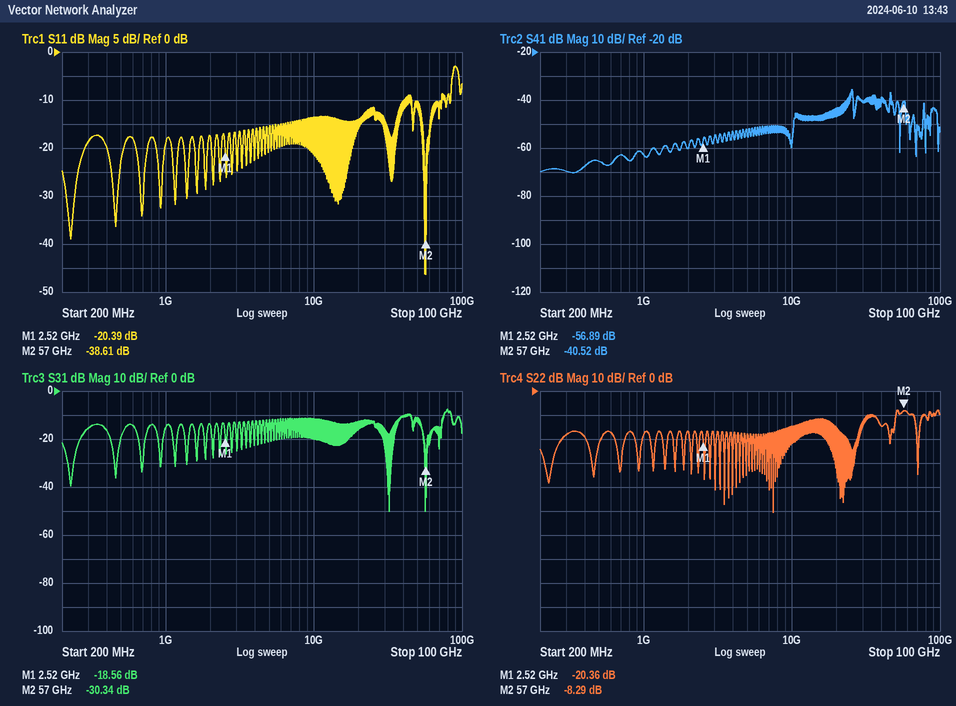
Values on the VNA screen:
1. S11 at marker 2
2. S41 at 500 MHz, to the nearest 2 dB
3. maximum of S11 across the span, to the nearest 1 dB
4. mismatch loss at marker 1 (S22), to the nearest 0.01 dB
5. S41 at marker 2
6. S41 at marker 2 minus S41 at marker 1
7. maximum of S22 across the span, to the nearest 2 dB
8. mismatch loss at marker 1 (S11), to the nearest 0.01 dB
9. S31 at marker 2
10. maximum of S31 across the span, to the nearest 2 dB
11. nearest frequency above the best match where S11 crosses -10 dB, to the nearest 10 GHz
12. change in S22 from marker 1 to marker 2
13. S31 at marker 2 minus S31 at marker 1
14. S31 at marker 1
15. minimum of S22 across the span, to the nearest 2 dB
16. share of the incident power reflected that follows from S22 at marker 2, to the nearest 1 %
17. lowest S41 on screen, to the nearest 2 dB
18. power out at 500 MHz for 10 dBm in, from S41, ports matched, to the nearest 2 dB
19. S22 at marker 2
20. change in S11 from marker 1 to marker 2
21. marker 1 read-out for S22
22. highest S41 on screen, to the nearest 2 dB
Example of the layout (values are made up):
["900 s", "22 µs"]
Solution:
["-38.61 dB", "-66 dB", "-3 dB", "0.04 dB", "-40.52 dB", "16.37 dB", "-8 dB", "0.04 dB", "-30.34 dB", "-8 dB", "70 GHz", "12.07 dB", "-11.78 dB", "-18.56 dB", "-50 dB", "15 %", "-70 dB", "-56 dBm", "-8.29 dB", "-18.22 dB", "-20.36 dB", "-36 dB"]
